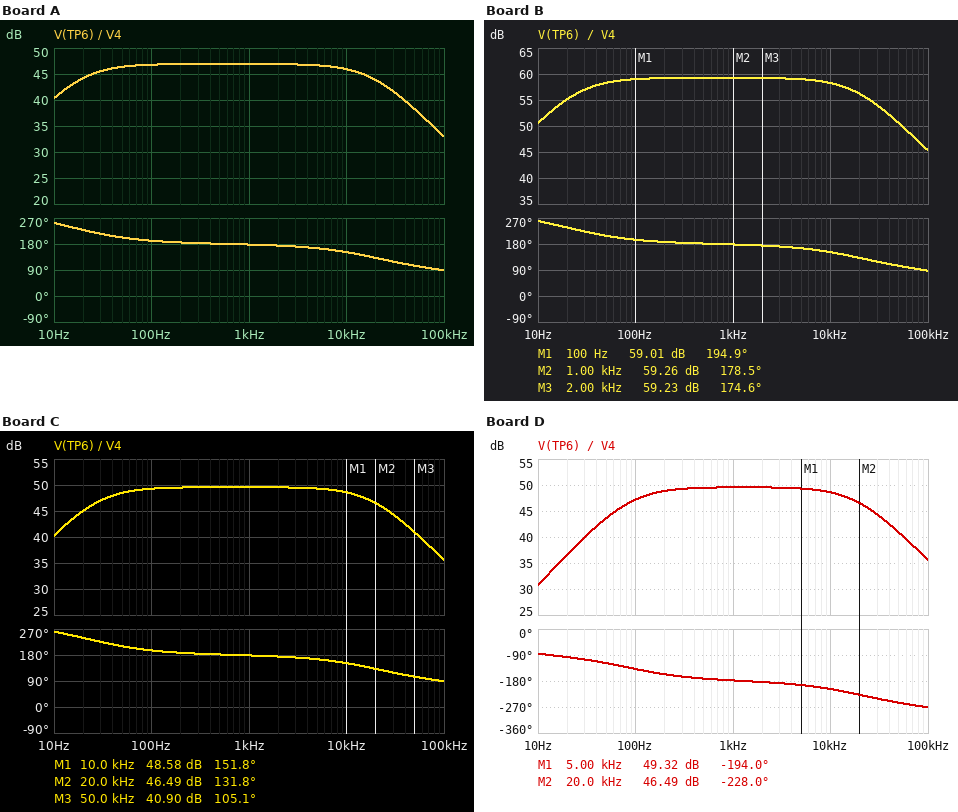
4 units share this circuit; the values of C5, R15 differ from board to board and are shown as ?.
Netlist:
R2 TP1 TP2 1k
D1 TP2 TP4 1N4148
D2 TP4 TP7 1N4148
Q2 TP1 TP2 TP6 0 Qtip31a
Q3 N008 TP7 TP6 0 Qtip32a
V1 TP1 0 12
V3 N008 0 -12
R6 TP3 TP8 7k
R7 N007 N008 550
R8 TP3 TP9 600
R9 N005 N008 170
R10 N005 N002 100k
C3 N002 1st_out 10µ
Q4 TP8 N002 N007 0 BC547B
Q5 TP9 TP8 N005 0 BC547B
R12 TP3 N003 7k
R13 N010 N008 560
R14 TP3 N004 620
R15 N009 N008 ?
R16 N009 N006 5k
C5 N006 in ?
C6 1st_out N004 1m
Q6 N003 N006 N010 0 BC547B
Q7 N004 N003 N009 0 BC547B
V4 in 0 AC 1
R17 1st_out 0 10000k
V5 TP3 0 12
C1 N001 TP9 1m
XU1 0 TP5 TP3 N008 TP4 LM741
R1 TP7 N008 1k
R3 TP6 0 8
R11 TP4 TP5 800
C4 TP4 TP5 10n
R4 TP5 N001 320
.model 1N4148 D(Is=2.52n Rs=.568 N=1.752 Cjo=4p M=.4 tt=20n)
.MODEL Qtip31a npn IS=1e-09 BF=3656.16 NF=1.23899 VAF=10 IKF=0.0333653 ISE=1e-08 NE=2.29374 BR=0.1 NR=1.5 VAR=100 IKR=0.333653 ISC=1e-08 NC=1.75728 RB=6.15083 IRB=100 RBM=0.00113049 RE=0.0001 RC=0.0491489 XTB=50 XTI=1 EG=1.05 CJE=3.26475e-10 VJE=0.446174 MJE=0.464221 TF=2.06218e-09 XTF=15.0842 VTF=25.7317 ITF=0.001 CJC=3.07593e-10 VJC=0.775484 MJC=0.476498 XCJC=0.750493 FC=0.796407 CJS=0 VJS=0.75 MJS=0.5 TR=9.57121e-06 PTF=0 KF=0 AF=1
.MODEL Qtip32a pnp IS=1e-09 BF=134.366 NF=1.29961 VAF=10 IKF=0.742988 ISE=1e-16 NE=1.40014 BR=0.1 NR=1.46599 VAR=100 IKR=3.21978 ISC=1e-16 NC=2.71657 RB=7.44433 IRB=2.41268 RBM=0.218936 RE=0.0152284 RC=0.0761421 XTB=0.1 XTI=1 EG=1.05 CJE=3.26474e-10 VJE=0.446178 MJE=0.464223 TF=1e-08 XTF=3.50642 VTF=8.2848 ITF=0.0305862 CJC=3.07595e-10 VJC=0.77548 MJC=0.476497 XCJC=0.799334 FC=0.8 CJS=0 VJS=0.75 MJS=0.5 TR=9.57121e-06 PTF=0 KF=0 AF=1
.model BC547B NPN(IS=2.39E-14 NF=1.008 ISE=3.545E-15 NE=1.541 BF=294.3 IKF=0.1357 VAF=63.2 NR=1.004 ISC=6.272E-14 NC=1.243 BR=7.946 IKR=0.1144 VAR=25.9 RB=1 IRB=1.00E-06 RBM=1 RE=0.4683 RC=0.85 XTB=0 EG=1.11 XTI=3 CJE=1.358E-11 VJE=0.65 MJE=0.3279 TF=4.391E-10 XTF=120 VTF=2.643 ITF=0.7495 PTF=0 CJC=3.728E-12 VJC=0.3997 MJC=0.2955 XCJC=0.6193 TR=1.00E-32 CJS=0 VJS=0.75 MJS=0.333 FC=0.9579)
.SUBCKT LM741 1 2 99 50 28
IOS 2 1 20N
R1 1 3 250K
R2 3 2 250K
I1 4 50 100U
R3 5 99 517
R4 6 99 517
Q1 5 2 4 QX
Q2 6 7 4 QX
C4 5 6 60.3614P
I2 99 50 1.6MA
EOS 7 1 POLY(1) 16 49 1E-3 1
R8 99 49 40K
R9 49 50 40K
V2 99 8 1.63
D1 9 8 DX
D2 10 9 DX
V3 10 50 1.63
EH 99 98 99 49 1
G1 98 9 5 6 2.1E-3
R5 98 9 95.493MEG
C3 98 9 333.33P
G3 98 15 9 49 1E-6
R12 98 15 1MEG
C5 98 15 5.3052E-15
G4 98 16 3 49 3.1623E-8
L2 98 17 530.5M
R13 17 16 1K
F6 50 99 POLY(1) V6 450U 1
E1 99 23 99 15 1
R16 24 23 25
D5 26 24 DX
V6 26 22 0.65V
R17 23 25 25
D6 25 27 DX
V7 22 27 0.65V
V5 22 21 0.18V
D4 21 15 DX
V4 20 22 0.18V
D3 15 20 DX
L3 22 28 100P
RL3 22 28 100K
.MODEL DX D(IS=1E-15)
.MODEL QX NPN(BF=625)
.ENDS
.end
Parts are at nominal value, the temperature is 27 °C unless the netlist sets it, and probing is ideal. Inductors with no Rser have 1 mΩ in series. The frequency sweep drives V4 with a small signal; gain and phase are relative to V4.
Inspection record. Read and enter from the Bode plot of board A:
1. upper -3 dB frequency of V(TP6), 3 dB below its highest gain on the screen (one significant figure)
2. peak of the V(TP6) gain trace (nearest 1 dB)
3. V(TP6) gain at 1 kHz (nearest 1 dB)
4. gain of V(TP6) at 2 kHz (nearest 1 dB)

20 kHz
47 dB
47 dB
47 dB
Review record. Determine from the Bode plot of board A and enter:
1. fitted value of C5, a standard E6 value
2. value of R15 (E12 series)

22 µF
1.2 kΩ
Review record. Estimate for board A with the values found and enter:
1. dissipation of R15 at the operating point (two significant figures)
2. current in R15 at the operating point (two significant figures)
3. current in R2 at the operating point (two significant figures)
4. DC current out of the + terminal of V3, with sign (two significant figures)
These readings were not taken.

4.8 mW
2.0 mA
11 mA
-560 mA
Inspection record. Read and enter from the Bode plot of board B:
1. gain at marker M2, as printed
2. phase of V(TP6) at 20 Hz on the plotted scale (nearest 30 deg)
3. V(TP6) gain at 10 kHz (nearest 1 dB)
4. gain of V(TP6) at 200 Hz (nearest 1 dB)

59.26 dB
240 deg
58 dB
59 dB
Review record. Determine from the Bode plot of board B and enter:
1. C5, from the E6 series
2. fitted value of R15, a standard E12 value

15 µF
220 Ω
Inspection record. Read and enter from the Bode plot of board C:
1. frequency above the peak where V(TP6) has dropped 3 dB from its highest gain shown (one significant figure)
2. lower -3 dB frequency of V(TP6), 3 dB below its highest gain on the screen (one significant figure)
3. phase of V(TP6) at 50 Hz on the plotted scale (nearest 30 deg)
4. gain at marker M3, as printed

20 kHz
30 Hz
210 deg
40.90 dB
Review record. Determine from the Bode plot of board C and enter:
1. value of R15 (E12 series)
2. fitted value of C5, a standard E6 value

820 Ω
15 µF
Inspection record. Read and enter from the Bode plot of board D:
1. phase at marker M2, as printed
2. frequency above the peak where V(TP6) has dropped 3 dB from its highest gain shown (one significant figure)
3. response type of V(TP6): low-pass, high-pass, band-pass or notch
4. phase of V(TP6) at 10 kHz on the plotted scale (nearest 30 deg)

-228.0 deg
20 kHz
band-pass
-210 deg
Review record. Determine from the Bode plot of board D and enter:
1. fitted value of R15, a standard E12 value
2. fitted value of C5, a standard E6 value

820 Ω
4.7 µF
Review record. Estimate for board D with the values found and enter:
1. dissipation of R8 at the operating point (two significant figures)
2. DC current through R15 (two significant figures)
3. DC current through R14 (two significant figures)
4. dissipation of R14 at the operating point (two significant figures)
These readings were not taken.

210 mW
2.9 mA
2.9 mA
5.3 mW
